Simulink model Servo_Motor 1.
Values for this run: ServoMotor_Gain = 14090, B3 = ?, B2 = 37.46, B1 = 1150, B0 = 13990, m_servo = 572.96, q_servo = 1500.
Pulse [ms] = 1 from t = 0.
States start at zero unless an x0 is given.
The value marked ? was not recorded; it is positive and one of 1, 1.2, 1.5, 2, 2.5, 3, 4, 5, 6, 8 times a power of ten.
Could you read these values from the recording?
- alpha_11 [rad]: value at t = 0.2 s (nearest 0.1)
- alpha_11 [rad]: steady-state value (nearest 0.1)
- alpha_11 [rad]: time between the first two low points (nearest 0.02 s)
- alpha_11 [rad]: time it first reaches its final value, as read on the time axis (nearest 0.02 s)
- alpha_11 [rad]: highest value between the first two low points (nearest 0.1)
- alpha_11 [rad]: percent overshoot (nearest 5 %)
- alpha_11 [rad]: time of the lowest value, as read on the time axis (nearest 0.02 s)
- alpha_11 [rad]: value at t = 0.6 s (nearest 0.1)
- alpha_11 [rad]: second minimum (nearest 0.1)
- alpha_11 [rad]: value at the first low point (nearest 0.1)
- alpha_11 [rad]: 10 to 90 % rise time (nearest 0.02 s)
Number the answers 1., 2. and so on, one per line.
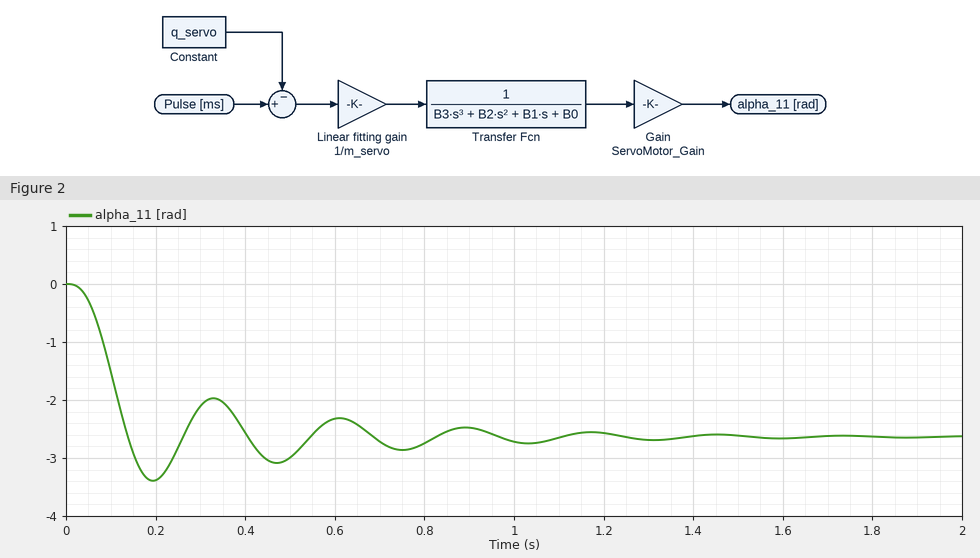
1. -3.4
2. -2.6
3. 0.28 s
4. 0.14 s
5. -2.0
6. 30 %
7. 0.20 s
8. -2.3
9. -3.1
10. -3.4
11. 0.08 s
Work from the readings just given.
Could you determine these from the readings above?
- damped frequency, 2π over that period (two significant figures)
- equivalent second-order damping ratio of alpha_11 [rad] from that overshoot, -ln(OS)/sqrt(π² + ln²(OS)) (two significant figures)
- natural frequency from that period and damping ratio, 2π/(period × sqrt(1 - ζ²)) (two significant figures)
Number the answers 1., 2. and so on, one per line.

1. 22 rad/s
2. 0.36
3. 24 rad/s
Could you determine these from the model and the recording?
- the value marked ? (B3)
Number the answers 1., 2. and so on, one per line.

1. 2
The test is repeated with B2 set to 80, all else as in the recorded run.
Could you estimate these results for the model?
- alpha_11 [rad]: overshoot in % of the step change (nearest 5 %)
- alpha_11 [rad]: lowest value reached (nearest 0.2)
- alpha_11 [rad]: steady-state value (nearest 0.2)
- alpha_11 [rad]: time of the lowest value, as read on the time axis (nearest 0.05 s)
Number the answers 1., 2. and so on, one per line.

1. 25 %
2. -3.2
3. -2.6
4. 0.25 s
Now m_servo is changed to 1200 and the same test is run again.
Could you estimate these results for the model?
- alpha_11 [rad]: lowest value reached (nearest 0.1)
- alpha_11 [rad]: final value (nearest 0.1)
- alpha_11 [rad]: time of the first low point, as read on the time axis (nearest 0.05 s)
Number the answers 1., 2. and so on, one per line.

1. -1.6
2. -1.3
3. 0.20 s
